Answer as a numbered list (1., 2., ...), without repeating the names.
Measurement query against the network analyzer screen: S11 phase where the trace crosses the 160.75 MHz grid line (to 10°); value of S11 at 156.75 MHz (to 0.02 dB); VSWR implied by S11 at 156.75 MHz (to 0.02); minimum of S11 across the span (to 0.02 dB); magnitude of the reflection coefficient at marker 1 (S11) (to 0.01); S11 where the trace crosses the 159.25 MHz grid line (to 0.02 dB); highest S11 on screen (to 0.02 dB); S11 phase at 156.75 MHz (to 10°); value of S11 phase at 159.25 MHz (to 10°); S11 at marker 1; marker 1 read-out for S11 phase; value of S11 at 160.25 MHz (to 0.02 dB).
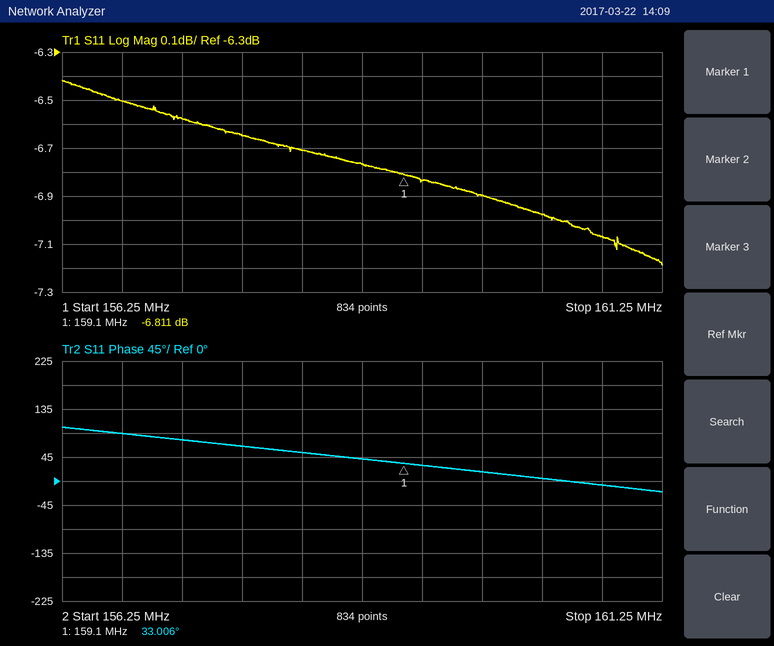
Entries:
1. -10°
2. -6.50 dB
3. 2.80
4. -7.18 dB
5. 0.46
6. -6.84 dB
7. -6.42 dB
8. 90°
9. 30°
10. -6.811 dB
11. 33.006°
12. -6.98 dB
